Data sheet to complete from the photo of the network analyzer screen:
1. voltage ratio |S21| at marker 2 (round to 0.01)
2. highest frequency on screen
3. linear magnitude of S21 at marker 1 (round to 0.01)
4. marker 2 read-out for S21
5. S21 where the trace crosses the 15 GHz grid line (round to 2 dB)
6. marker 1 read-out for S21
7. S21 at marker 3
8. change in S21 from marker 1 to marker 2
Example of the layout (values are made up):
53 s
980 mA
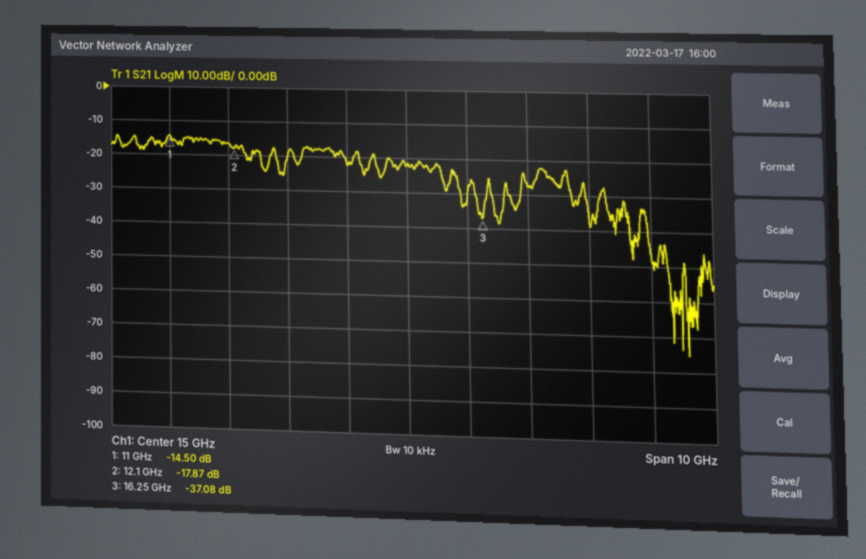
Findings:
0.13
20 GHz
0.19
-17.87 dB
-22 dB
-14.50 dB
-37.08 dB
-3.37 dB
